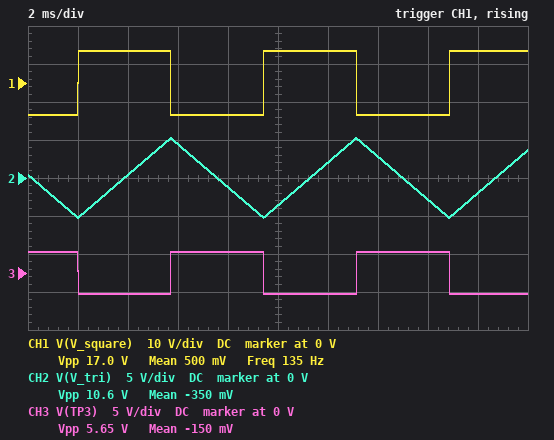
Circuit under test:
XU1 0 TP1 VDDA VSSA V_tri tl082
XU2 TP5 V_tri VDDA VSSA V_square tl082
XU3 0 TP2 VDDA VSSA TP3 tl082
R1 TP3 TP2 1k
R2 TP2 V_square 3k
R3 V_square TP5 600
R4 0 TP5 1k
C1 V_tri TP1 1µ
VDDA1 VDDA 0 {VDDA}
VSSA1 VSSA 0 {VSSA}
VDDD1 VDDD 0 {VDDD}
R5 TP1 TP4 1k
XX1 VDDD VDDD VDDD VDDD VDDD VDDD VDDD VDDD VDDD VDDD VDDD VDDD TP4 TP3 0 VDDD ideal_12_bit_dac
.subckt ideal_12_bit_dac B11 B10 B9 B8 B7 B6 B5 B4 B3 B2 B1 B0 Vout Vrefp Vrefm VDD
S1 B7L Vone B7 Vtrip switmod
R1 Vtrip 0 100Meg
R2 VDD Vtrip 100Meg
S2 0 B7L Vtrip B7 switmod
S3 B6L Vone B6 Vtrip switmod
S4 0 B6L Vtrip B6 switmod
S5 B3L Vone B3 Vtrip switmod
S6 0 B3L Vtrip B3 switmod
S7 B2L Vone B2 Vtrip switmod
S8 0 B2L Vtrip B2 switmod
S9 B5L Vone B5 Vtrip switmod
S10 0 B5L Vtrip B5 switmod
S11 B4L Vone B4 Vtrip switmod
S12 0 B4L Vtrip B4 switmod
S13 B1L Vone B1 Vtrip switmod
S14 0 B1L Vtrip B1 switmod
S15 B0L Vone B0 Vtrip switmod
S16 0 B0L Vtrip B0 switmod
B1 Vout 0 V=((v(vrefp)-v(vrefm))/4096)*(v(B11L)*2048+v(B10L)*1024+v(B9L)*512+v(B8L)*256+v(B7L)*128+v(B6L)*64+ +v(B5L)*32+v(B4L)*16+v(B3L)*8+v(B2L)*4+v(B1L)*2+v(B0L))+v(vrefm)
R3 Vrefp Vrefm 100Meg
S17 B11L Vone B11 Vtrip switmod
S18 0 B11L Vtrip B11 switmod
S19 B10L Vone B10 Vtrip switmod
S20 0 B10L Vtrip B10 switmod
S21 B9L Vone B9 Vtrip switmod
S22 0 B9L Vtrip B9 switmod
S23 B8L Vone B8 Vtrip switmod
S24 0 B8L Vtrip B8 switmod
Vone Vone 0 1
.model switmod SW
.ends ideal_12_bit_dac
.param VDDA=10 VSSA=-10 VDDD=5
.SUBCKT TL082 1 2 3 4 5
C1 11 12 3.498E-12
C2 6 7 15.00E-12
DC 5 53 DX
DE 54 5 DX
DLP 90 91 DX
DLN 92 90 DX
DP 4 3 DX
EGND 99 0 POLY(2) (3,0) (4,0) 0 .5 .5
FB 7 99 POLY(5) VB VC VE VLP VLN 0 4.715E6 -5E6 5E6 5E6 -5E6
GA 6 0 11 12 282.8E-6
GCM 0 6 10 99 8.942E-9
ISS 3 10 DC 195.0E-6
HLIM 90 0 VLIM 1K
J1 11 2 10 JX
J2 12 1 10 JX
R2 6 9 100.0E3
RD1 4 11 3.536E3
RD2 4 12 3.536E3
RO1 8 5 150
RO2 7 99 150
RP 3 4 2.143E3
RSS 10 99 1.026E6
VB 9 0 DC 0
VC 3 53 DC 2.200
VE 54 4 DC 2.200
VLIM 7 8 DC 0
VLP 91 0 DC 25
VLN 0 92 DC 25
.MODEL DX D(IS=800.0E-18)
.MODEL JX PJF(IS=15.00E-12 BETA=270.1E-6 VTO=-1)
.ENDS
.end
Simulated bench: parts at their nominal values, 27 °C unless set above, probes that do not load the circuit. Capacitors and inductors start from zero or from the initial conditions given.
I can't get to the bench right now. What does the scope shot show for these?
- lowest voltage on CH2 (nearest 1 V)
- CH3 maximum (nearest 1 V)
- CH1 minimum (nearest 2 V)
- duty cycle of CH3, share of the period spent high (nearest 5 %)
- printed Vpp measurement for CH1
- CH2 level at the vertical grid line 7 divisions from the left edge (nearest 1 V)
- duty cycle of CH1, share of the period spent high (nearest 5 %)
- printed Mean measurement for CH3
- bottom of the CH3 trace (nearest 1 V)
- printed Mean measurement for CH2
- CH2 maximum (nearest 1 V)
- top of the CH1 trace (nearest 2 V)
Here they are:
-5 V
3 V
-8 V
50 %
17.0 V
3 V
50 %
-150 mV
-3 V
-350 mV
5 V
8 V
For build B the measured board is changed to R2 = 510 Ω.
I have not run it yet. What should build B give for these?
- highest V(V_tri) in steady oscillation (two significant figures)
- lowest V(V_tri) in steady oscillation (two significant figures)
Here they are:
5.4 V
-5.4 V
